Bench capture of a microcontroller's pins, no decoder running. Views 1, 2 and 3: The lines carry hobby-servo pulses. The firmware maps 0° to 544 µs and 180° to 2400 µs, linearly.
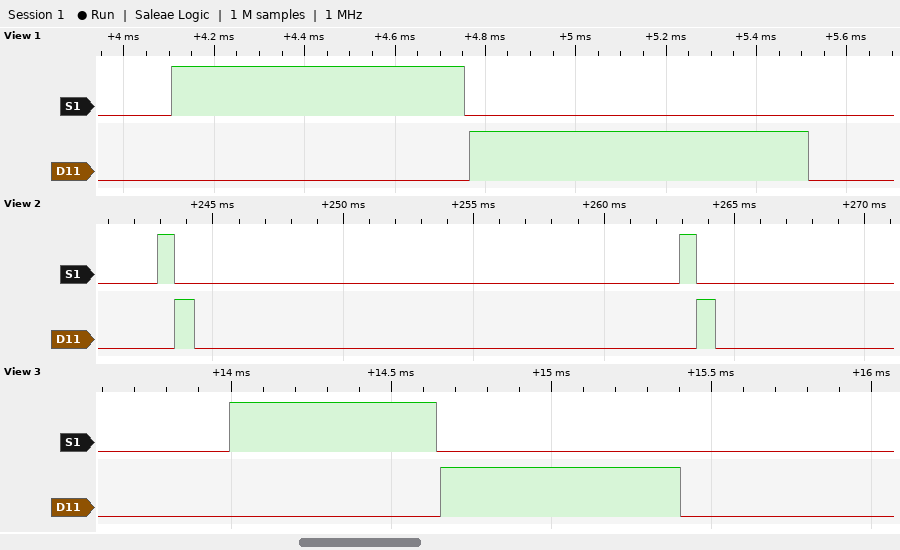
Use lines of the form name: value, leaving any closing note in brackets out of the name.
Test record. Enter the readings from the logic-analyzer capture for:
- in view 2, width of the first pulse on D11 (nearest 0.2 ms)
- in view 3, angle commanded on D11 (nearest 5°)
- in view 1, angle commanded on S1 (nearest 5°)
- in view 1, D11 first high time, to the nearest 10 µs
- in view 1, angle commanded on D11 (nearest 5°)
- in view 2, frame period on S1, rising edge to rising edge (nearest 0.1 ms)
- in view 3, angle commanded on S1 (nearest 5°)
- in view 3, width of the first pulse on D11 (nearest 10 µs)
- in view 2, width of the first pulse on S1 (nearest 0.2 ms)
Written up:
in view 2, width of the first pulse on D11: 0.8 ms
in view 3, angle commanded on D11: 20°
in view 1, angle commanded on S1: 10°
in view 1, D11 first high time, to the nearest 10 µs: 750 µs
in view 1, angle commanded on D11: 20°
in view 2, frame period on S1, rising edge to rising edge: 20.0 ms
in view 3, angle commanded on S1: 10°
in view 3, width of the first pulse on D11: 750 µs
in view 2, width of the first pulse on S1: 0.6 ms
